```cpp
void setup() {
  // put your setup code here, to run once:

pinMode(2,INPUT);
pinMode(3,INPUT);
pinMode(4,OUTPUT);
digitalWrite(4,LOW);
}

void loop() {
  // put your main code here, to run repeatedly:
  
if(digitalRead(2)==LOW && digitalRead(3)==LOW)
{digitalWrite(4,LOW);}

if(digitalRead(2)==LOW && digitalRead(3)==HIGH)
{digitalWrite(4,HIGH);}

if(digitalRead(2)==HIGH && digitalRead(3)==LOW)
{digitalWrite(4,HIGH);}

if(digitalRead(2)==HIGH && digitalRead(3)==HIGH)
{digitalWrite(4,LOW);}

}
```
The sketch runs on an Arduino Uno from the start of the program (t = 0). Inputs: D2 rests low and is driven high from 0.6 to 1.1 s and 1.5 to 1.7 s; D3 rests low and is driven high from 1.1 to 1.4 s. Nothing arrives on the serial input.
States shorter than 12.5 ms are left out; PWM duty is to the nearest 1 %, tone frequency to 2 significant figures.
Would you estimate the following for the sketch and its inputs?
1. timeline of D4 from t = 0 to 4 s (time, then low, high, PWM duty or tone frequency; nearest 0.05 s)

0 s low; 0.6 s high; 1.4 s low; 1.5 s high; 1.7 s low
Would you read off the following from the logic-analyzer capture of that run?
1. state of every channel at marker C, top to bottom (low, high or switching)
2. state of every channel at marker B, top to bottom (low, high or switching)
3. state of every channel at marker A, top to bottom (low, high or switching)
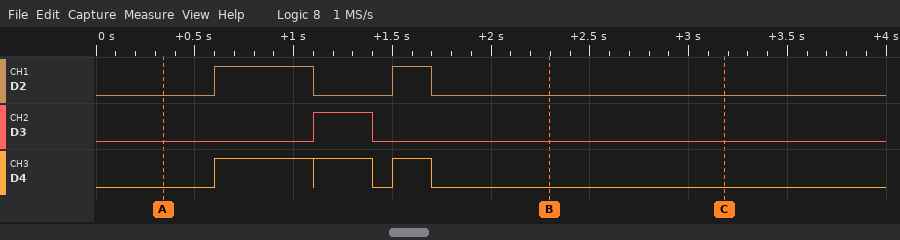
D2 low, D3 low, D4 low
D2 low, D3 low, D4 low
D2 low, D3 low, D4 low
